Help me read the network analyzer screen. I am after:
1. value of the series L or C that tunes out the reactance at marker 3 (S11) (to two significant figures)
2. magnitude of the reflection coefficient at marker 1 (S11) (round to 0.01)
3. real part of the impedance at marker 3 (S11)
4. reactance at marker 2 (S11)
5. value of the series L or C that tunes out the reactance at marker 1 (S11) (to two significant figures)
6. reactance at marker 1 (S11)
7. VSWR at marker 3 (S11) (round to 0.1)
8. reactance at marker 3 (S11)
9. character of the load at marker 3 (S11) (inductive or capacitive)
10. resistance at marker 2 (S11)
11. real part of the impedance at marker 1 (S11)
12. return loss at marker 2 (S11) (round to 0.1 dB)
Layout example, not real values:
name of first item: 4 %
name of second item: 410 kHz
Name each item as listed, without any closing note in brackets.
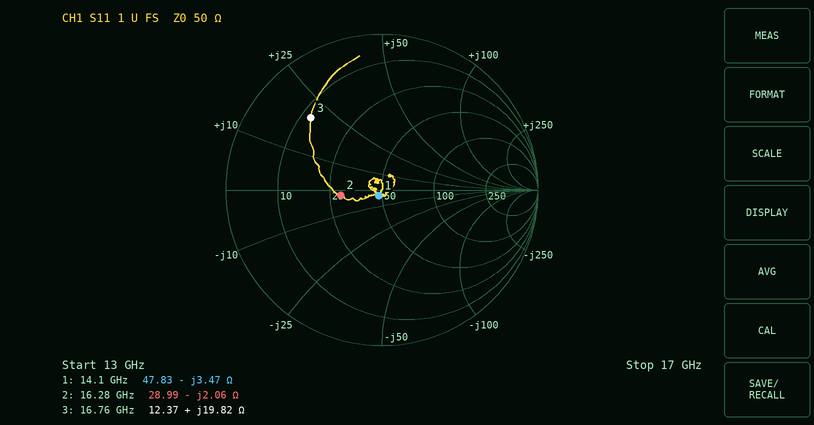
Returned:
value of the series L or C that tunes out the reactance at marker 3 (S11): 480 fF
magnitude of the reflection coefficient at marker 1 (S11): 0.04
real part of the impedance at marker 3: 12.37 Ω
reactance at marker 2: -2.06 Ω
value of the series L or C that tunes out the reactance at marker 1 (S11): 39 pH
reactance at marker 1: -3.47 Ω
VSWR at marker 3 (S11): 4.7
reactance at marker 3: +19.82 Ω
character of the load at marker 3 (S11): inductive
resistance at marker 2: 28.99 Ω
real part of the impedance at marker 1: 47.83 Ω
return loss at marker 2 (S11): 11.5 dB
